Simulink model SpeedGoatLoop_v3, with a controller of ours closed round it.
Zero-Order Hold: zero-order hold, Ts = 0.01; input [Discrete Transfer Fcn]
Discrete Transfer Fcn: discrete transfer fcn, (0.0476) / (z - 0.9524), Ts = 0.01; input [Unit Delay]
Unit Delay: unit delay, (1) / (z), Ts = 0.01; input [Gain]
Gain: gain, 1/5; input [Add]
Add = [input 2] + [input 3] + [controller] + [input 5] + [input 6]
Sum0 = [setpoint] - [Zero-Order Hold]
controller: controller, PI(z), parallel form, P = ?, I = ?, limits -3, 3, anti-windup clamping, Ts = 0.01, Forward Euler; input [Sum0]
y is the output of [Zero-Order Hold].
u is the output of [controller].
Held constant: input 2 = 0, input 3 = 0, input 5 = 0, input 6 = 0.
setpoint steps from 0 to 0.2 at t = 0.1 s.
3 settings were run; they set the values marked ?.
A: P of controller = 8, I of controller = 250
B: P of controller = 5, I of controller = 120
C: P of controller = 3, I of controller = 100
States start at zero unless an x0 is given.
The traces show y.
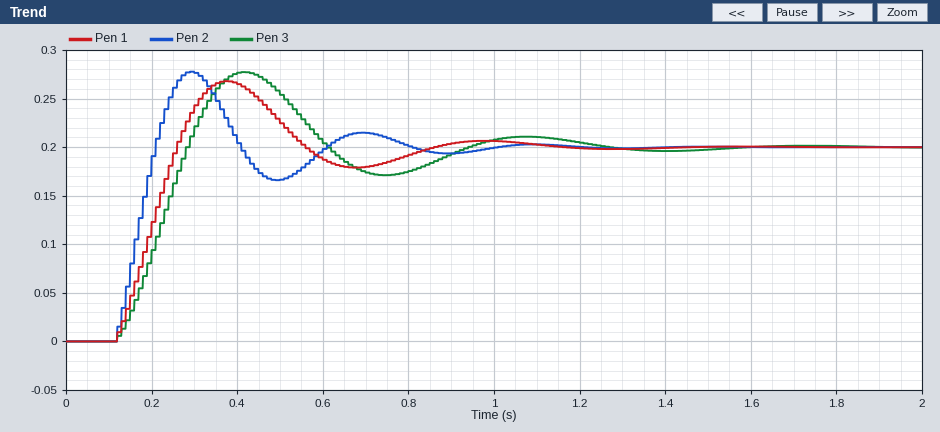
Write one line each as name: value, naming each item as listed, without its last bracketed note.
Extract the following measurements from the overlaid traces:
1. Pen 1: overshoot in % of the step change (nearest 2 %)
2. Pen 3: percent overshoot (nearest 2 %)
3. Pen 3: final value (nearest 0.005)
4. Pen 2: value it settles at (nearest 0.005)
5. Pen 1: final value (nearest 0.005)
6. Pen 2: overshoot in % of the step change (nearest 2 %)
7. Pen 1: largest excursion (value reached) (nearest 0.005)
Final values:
Pen 1: overshoot in % of the step change: 34 %
Pen 3: percent overshoot: 38 %
Pen 3: final value: 0.200
Pen 2: value it settles at: 0.200
Pen 1: final value: 0.200
Pen 2: overshoot in % of the step change: 38 %
Pen 1: largest excursion (value reached): 0.270
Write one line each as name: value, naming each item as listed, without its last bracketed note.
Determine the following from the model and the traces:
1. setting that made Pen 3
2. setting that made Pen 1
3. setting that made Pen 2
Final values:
setting that made Pen 3: C
setting that made Pen 1: B
setting that made Pen 2: A
